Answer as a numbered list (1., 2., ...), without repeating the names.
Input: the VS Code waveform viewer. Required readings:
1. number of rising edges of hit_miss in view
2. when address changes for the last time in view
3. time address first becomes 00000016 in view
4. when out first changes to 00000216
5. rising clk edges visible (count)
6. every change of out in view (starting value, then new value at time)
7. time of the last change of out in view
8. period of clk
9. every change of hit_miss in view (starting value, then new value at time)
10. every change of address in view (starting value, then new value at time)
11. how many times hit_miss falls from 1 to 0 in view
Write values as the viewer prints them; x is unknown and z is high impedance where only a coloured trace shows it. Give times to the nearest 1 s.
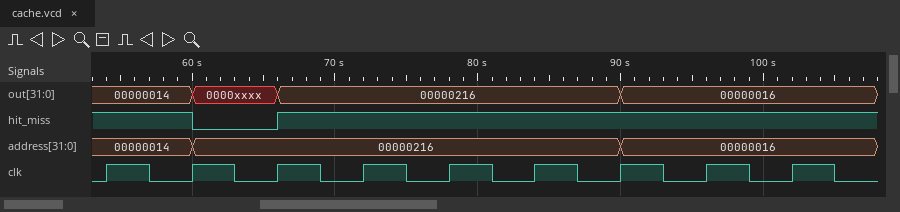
1. 1
2. 90 s
3. 90 s
4. 66 s
5. 9
6. 00000014, 0000xxxx at 60 s, 00000216 at 66 s, 00000016 at 90 s
7. 90 s
8. 6 s
9. 1, 0 at 60 s, 1 at 66 s
10. 00000014, 00000216 at 60 s, 00000016 at 90 s
11. 1
